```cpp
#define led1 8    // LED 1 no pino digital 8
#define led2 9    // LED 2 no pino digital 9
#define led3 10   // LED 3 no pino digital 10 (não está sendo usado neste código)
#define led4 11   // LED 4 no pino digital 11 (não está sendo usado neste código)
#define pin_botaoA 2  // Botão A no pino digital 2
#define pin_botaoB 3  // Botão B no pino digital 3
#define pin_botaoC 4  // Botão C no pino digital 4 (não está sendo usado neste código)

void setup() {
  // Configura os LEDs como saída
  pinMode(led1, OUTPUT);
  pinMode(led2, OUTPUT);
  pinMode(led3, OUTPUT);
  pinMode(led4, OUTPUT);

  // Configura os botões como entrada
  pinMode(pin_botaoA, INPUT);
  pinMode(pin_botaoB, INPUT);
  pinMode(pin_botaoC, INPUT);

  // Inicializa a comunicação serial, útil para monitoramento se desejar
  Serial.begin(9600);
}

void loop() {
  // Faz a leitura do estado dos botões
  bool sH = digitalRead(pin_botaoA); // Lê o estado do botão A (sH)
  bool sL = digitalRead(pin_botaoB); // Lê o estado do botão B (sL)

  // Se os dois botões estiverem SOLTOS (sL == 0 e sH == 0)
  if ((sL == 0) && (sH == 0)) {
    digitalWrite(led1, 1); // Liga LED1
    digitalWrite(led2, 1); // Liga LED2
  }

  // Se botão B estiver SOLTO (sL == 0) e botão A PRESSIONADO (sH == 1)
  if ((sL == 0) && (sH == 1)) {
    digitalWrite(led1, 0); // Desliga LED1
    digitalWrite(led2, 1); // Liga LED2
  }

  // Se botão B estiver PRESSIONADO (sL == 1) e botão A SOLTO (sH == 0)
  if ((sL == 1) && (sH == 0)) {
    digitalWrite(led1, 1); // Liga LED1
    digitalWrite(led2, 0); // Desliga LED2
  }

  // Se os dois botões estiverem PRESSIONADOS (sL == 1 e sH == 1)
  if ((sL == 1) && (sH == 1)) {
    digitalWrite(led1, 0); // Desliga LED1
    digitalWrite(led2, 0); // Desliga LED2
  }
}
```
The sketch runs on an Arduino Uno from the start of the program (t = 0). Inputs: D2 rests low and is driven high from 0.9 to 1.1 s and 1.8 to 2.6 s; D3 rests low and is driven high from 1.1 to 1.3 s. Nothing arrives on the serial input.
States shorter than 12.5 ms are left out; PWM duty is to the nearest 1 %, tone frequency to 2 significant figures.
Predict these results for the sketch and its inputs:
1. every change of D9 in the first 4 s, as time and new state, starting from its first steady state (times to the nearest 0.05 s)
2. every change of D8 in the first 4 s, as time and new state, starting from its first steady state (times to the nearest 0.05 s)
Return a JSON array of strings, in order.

["0 s high; 1.1 s low; 1.3 s high", "0 s high; 0.9 s low; 1.1 s high; 1.8 s low; 2.6 s high"]
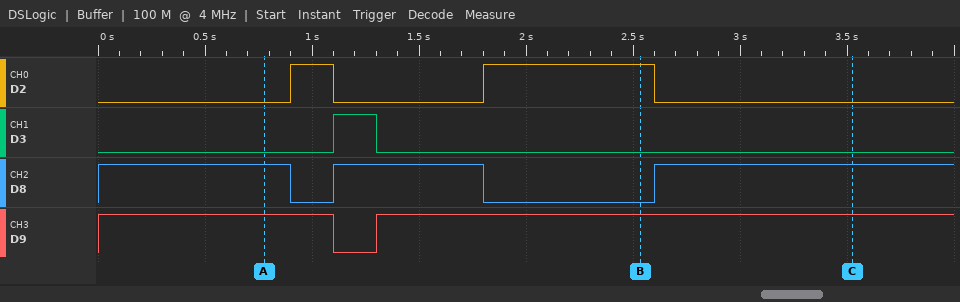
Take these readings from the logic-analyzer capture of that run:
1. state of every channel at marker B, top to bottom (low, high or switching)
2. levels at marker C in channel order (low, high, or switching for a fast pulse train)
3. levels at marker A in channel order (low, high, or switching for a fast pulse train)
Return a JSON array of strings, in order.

["D2 high, D3 low, D8 low, D9 high", "D2 low, D3 low, D8 high, D9 high", "D2 low, D3 low, D8 high, D9 high"]
